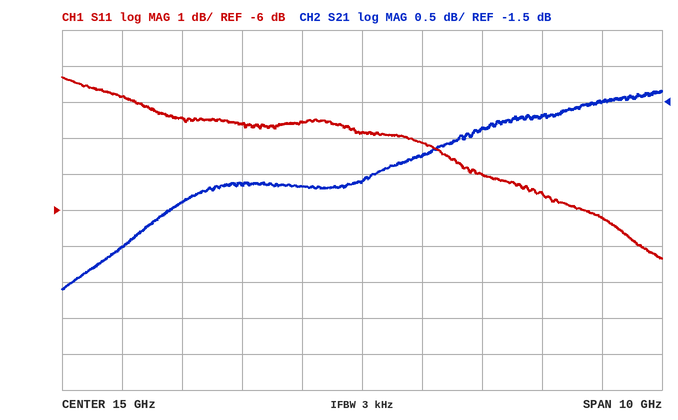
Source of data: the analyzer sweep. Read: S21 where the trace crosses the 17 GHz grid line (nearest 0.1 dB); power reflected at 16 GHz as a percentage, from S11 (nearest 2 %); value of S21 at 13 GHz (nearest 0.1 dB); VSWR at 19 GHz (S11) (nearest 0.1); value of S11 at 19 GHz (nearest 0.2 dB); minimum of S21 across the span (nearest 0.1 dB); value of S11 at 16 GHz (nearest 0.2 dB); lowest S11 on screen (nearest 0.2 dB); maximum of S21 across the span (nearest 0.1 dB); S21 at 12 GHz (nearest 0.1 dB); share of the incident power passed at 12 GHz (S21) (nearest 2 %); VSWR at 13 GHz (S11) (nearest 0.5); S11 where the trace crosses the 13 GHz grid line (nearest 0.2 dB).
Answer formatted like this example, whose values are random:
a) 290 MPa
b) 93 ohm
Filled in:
a) -1.9 dB
b) 38 %
c) -2.6 dB
d) 2.9
e) -6.2 dB
f) -4.1 dB
g) -4.2 dB
h) -7.4 dB
i) -1.3 dB
j) -2.9 dB
k) 52 %
l) 5.0
m) -3.6 dB
